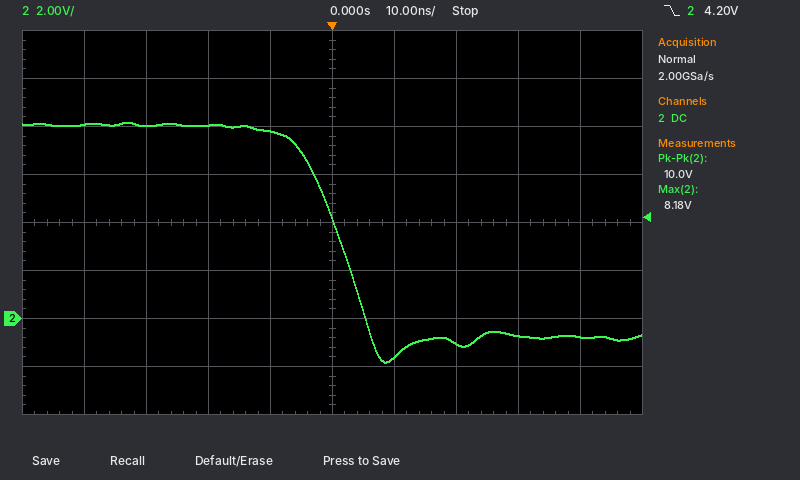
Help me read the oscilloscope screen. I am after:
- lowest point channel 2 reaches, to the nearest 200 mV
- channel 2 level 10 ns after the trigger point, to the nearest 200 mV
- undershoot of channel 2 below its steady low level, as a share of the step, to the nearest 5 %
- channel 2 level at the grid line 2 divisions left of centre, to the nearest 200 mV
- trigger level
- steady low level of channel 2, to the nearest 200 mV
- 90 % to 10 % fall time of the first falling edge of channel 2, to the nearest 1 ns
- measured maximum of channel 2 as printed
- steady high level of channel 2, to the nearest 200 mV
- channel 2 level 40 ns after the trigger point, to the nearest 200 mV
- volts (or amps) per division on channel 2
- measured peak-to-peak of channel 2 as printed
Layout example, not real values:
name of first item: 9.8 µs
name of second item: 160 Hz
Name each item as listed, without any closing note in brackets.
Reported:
lowest point channel 2 reaches, to the nearest 200 mV: -1.8 V
channel 2 level 10 ns after the trigger point, to the nearest 200 mV: -1.6 V
undershoot of channel 2 below its steady low level, as a share of the step, to the nearest 5 %: 10 %
channel 2 level at the grid line 2 divisions left of centre, to the nearest 200 mV: 8.0 V
trigger level: 4.20 V
steady low level of channel 2, to the nearest 200 mV: -800 mV
90 % to 10 % fall time of the first falling edge of channel 2, to the nearest 1 ns: 11 ns
measured maximum of channel 2 as printed: 8.18 V
steady high level of channel 2, to the nearest 200 mV: 8.0 V
channel 2 level 40 ns after the trigger point, to the nearest 200 mV: -800 mV
volts (or amps) per division on channel 2: 2 V
measured peak-to-peak of channel 2 as printed: 10.0 V
